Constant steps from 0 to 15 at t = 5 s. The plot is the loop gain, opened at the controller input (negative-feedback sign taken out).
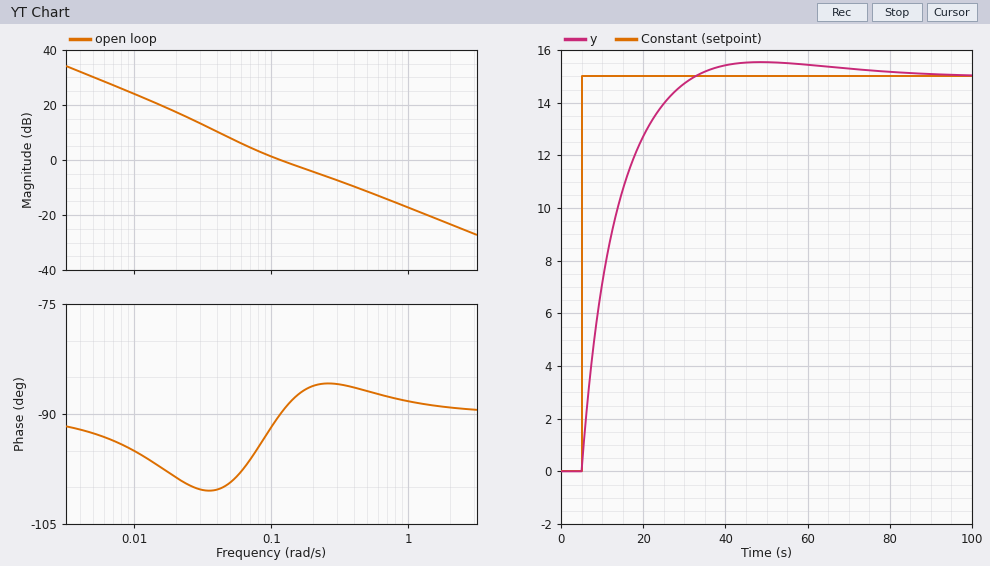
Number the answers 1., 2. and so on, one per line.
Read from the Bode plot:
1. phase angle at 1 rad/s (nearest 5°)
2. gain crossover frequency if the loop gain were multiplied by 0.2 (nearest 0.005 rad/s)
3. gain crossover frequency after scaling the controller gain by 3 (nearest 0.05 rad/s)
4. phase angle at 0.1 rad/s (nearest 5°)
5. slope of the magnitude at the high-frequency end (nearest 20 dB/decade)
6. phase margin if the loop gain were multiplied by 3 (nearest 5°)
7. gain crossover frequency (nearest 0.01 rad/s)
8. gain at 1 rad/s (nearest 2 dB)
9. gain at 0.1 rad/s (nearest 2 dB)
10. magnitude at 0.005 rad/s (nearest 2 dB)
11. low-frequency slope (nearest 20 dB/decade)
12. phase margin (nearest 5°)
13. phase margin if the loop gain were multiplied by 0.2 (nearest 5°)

1. -90°
2. 0.030 rad/s
3. 0.40 rad/s
4. -90°
5. -20 dB/decade
6. 95°
7. 0.12 rad/s
8. -18 dB
9. 2 dB
10. 30 dB
11. -20 dB/decade
12. 90°
13. 80°
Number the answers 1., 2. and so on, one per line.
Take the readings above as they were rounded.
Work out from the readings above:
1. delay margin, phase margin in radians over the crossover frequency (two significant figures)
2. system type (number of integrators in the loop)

1. 13 s
2. 1
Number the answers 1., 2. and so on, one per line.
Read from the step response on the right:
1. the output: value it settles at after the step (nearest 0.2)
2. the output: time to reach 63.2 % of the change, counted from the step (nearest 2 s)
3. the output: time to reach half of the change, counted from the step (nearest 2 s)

1. 15.0
2. 8 s
3. 6 s
